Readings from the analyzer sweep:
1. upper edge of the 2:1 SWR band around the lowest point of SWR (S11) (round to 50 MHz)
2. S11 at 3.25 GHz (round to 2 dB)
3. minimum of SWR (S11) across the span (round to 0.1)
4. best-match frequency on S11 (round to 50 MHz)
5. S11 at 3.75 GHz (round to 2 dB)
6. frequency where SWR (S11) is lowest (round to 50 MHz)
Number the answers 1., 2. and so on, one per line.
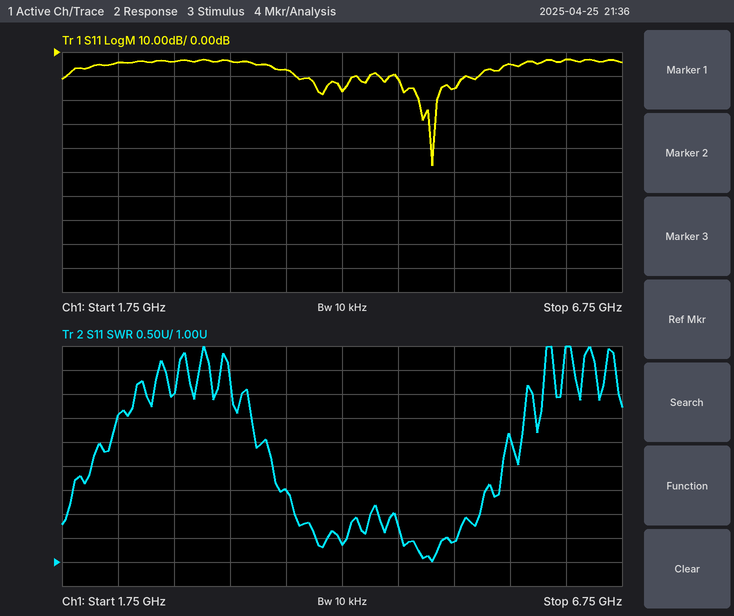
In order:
1. 5.50 GHz
2. -4 dB
3. 1.0
4. 5.05 GHz
5. -8 dB
6. 5.05 GHz
